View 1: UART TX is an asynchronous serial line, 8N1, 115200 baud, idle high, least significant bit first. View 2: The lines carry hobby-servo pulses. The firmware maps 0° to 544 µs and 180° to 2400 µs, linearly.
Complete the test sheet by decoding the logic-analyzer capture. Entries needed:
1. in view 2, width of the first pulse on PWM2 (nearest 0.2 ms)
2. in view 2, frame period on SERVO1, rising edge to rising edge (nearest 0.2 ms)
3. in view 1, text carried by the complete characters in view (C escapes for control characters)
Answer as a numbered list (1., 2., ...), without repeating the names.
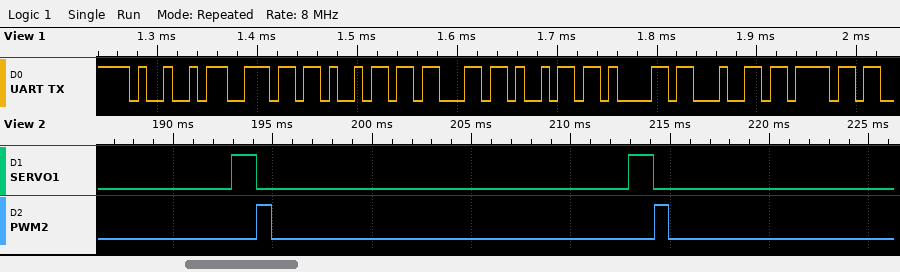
1. 0.8 ms
2. 20.0 ms
3. "Iniciado"
